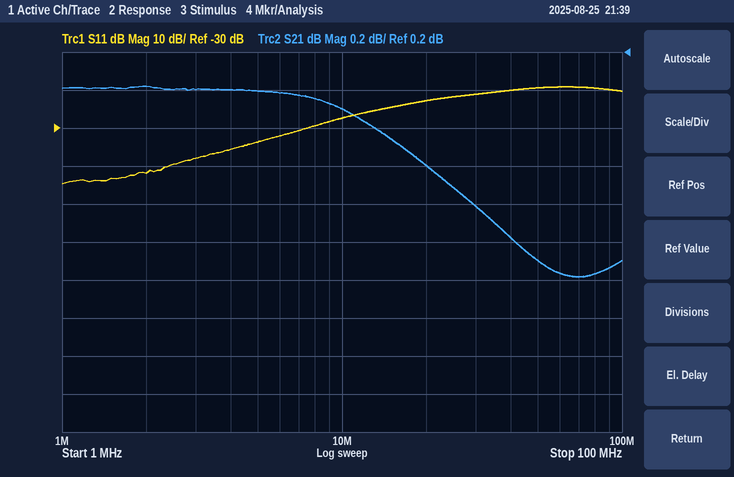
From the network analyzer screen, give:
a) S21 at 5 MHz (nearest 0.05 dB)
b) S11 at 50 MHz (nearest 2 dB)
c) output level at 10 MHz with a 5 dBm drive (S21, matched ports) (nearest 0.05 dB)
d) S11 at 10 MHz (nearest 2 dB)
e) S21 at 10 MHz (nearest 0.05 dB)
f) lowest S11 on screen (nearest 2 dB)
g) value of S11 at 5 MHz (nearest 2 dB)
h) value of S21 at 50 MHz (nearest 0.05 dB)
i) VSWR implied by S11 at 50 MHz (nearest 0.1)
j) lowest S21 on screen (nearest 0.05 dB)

0.00 dB
-20 dB
4.90 dBm
-28 dB
-0.10 dB
-44 dB
-34 dB
-0.90 dB
1.2
-1.00 dB
